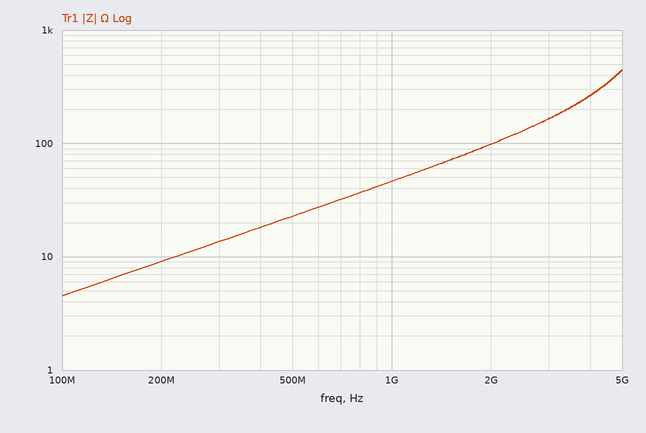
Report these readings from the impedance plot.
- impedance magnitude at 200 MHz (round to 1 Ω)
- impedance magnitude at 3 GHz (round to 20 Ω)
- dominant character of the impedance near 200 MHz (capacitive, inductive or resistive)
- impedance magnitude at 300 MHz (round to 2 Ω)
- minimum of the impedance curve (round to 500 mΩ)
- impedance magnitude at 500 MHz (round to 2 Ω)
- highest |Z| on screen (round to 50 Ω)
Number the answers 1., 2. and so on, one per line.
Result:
1. 9 Ω
2. 160 Ω
3. inductive
4. 14 Ω
5. 4.5 Ω
6. 22 Ω
7. 450 Ω
